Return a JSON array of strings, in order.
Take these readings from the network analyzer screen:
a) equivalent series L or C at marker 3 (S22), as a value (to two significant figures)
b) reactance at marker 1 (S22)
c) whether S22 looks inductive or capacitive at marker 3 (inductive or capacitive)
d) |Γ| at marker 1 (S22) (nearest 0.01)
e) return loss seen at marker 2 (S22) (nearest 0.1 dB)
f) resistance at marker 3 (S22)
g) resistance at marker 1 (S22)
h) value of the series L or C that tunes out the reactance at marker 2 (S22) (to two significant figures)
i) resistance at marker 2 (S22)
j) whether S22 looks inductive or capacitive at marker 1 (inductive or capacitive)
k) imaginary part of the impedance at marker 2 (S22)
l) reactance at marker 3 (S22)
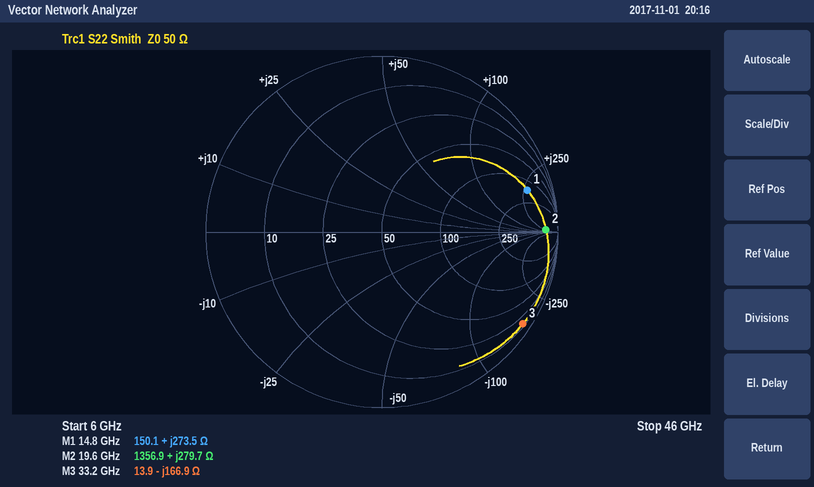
["29 fF", "+273.5 Ω", "capacitive", "0.86", "0.6 dB", "13.9 Ω", "150.1 Ω", "29 fF", "1356.9 Ω", "inductive", "+279.7 Ω", "-166.9 Ω"]
